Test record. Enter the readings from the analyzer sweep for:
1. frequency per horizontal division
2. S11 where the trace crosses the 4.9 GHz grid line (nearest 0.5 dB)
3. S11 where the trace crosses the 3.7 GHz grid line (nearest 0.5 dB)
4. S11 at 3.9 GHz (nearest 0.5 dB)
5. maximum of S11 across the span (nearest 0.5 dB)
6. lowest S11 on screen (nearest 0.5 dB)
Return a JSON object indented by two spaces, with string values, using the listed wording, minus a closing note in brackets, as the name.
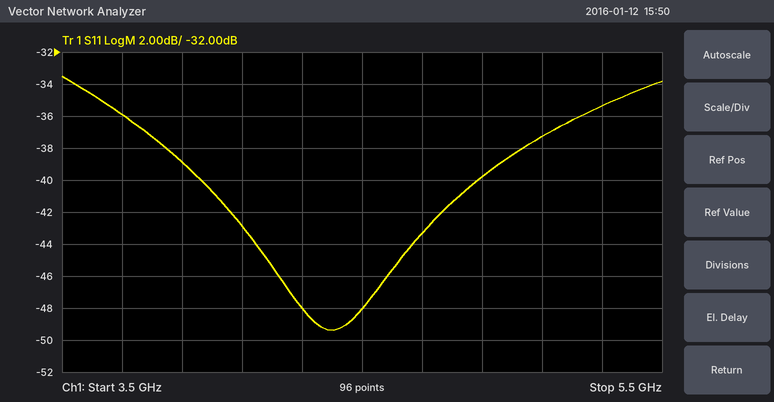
{
  "frequency per horizontal division": "200 MHz",
  "S11 where the trace crosses the 4.9 GHz grid line": "-40.0 dB",
  "S11 where the trace crosses the 3.7 GHz grid line": "-36.0 dB",
  "S11 at 3.9 GHz": "-39.0 dB",
  "maximum of S11 across the span": "-33.5 dB",
  "lowest S11 on screen": "-49.5 dB"
}
